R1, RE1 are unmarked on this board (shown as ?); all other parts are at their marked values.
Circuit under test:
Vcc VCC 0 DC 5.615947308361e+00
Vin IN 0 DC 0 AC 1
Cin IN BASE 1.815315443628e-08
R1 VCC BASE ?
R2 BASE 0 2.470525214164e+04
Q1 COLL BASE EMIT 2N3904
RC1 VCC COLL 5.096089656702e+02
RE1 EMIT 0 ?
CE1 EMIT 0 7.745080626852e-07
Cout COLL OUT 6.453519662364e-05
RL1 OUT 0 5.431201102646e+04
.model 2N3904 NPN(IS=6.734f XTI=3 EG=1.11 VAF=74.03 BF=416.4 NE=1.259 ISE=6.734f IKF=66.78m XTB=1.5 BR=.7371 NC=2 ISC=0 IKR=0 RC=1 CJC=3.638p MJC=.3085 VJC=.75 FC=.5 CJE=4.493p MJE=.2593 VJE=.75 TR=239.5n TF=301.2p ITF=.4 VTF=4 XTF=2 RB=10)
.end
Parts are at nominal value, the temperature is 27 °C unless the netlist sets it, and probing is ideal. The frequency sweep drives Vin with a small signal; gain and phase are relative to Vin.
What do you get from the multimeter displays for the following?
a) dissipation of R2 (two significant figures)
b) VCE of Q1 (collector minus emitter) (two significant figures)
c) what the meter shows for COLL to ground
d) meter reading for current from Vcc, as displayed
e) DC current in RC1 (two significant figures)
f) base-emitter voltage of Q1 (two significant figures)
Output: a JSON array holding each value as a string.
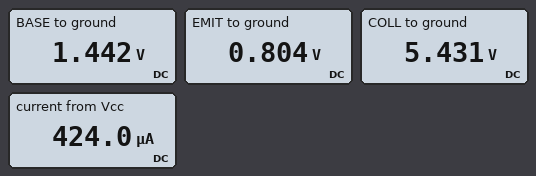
["84 µW", "4.6 V", "5.431 V", "424.0 µA", "360 µA", "640 mV"]
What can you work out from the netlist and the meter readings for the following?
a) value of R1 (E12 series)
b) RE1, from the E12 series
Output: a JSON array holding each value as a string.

["68 kΩ", "2.2 kΩ"]
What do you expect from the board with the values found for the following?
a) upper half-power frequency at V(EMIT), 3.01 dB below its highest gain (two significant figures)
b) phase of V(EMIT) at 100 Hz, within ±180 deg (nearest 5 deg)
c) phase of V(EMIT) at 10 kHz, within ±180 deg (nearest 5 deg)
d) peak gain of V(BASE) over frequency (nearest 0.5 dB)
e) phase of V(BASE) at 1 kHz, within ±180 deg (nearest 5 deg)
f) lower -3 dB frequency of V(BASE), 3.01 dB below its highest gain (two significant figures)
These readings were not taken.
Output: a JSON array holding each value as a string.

["4.6 kHz", "75 deg", "-65 deg", "0 dB", "25 deg", "890 Hz"]
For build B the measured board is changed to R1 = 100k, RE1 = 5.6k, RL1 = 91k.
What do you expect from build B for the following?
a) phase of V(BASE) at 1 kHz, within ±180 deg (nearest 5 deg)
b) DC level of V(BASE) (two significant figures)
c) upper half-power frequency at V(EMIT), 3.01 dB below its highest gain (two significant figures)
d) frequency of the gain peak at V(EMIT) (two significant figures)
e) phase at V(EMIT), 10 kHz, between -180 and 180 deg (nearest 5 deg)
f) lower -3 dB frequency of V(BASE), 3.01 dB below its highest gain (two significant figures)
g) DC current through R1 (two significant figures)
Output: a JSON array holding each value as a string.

["30 deg", "1.1 V", "1.6 kHz", "580 Hz", "-80 deg", "720 Hz", "45 µA"]
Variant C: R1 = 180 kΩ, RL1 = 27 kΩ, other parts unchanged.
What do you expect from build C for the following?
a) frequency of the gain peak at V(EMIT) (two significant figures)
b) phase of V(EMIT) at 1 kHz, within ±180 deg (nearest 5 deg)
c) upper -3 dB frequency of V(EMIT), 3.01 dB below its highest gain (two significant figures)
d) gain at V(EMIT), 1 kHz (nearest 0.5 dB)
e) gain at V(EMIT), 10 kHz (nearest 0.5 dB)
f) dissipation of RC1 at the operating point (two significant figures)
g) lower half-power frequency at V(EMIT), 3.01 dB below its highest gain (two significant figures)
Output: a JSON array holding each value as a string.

["420 Hz", "-40 deg", "1.1 kHz", "-12.0 dB", "-30.0 dB", "790 nW", "160 Hz"]
